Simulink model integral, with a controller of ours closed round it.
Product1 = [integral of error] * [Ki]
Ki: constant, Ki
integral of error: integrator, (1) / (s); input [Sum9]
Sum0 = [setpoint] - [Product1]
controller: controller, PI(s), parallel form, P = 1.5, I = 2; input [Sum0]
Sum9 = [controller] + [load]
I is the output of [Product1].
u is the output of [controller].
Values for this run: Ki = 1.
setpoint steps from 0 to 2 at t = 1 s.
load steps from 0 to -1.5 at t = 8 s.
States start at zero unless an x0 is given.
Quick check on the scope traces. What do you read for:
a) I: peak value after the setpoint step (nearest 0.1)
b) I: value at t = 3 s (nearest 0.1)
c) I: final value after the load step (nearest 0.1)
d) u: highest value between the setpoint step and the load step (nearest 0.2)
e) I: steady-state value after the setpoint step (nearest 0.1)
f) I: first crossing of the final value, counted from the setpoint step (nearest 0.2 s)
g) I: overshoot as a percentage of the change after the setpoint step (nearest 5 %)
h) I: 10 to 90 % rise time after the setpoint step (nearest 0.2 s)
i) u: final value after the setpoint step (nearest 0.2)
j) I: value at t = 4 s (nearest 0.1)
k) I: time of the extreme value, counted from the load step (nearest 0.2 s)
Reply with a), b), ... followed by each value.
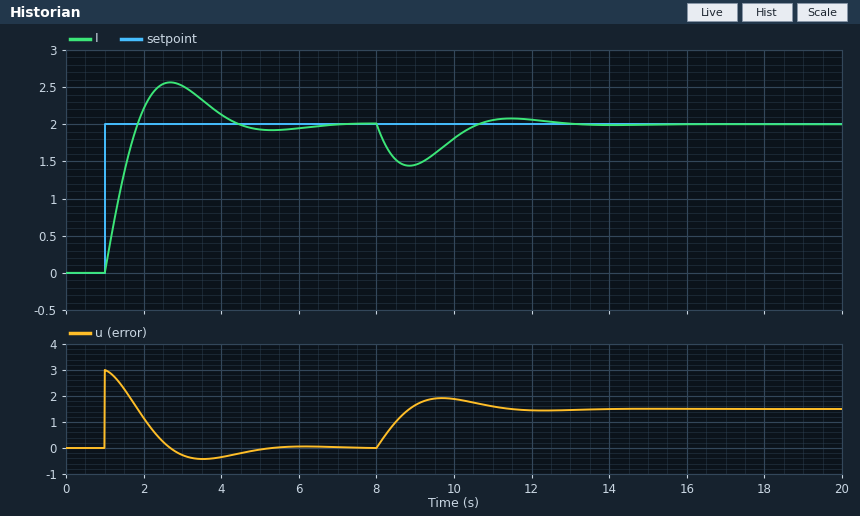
a) 2.6
b) 2.5
c) 2.0
d) 3.0
e) 2.0
f) 0.8 s
g) 30 %
h) 0.6 s
i) 0.0
j) 2.1
k) 0.8 s
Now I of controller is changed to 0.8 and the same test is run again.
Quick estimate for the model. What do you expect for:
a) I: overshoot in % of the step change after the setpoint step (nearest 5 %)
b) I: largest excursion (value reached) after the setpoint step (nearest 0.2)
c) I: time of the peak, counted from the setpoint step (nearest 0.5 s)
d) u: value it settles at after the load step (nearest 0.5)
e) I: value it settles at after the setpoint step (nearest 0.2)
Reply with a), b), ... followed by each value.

a) 15 %
b) 2.4
c) 2.5 s
d) 1.5
e) 2.0
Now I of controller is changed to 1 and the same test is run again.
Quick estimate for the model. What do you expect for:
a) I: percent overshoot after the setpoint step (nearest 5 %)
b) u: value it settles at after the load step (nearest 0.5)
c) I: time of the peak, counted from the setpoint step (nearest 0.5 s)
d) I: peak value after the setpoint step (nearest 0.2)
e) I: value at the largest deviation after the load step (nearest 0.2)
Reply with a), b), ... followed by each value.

a) 20 %
b) 1.5
c) 2.0 s
d) 2.4
e) 1.4
